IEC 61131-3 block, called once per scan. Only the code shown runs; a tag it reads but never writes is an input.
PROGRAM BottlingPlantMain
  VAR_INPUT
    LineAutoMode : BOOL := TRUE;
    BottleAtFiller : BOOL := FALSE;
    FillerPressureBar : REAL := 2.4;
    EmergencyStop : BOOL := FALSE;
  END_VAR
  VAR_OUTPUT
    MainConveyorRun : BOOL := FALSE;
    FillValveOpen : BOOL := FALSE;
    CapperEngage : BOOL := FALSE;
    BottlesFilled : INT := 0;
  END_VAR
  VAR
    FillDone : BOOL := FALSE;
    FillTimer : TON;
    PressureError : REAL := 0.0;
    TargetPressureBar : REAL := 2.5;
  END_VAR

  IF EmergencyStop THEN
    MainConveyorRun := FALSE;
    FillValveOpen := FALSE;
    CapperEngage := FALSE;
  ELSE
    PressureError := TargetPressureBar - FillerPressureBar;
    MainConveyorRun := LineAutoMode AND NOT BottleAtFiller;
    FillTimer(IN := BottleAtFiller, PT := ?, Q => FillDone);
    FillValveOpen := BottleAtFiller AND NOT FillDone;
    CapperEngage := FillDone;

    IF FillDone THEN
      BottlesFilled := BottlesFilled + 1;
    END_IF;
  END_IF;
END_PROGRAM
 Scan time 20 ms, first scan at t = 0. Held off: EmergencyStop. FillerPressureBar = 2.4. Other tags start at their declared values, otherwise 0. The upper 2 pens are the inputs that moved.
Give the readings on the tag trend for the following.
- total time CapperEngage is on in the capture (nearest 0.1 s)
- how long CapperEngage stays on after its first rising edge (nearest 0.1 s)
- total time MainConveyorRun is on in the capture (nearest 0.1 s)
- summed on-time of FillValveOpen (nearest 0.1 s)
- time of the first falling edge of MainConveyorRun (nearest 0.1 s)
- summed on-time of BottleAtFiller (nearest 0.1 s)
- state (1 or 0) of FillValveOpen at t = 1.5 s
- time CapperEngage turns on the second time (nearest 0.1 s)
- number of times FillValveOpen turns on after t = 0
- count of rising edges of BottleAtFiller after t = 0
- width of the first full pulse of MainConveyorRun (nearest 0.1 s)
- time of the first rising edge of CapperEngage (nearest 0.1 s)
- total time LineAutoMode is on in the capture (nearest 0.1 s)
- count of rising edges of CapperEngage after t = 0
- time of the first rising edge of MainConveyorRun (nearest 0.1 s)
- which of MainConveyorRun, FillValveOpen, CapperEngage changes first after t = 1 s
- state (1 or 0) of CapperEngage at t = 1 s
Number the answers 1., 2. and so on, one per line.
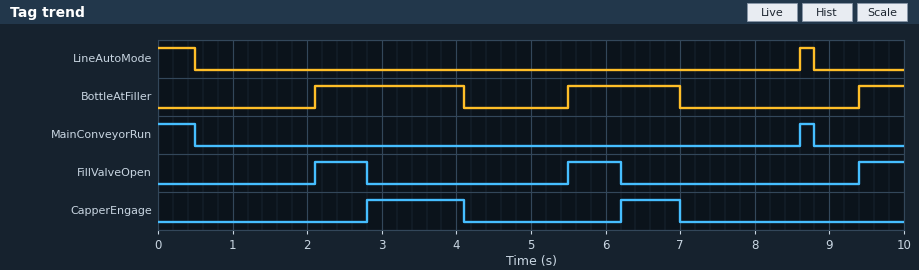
1. 2.1 s
2. 1.3 s
3. 0.7 s
4. 2.0 s
5. 0.5 s
6. 4.1 s
7. 0
8. 6.2 s
9. 3
10. 3
11. 0.2 s
12. 2.8 s
13. 0.7 s
14. 2
15. 8.6 s
16. FillValveOpen
17. 0
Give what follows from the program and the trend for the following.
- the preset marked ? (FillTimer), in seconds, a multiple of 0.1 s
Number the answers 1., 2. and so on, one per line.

1. 0.7 s
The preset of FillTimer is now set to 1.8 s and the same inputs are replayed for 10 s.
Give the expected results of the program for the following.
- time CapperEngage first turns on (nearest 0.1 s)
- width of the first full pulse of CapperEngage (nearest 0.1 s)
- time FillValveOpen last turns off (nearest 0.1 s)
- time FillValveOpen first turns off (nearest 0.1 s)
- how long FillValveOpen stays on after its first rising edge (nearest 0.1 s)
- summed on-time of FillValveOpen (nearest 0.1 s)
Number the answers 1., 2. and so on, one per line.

1. 3.9 s
2. 0.2 s
3. 7.0 s
4. 3.9 s
5. 1.8 s
6. 3.9 s
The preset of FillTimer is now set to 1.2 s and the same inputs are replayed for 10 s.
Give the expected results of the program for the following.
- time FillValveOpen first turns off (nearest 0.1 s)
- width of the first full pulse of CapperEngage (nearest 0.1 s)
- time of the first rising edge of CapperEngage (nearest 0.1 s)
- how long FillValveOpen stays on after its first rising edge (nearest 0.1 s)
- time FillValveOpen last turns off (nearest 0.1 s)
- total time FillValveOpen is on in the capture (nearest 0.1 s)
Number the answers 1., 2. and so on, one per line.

1. 3.3 s
2. 0.8 s
3. 3.3 s
4. 1.2 s
5. 6.7 s
6. 3.0 s
